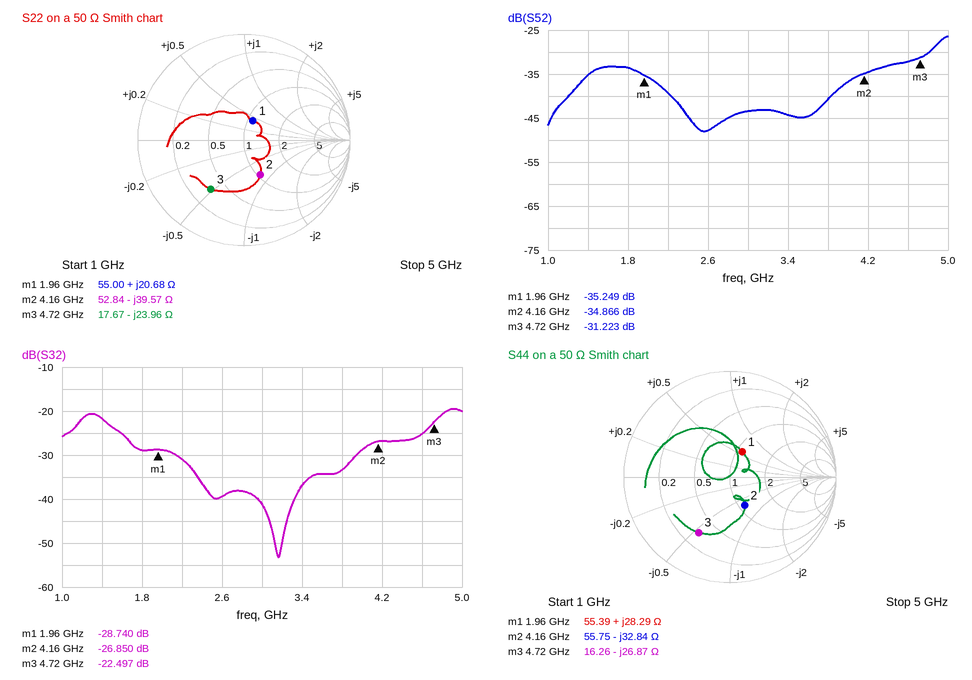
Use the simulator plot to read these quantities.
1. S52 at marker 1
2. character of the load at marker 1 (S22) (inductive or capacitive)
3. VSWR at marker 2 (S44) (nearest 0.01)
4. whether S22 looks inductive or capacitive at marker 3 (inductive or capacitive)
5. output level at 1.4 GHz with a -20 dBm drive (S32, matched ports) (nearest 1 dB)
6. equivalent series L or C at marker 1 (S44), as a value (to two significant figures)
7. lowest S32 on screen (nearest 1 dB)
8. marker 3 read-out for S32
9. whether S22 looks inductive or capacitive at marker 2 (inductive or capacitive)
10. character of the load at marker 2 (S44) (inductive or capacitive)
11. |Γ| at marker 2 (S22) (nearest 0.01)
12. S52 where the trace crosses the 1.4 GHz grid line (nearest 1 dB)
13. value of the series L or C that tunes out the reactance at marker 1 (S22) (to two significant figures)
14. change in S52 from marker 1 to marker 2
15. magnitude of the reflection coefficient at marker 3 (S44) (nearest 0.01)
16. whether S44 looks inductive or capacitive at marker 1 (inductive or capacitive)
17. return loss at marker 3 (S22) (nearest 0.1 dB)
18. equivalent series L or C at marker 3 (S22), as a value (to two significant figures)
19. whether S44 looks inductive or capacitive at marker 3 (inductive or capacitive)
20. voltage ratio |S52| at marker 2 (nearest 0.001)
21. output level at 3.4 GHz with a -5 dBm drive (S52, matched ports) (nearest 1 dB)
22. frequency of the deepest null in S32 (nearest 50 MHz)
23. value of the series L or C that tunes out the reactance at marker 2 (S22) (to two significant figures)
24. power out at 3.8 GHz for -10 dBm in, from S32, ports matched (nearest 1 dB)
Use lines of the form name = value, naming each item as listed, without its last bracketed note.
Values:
S52 at marker 1 = -35.249 dB
character of the load at marker 1 (S22) = inductive
VSWR at marker 2 (S44) = 1.86
whether S22 looks inductive or capacitive at marker 3 = capacitive
output level at 1.4 GHz with a -20 dBm drive (S32, matched ports) = -42 dBm
equivalent series L or C at marker 1 (S44), as a value = 2.3 nH
lowest S32 on screen = -53 dB
marker 3 read-out for S32 = -22.497 dB
whether S22 looks inductive or capacitive at marker 2 = capacitive
character of the load at marker 2 (S44) = capacitive
|Γ| at marker 2 (S22) = 0.36
S52 where the trace crosses the 1.4 GHz grid line = -35 dB
value of the series L or C that tunes out the reactance at marker 1 (S22) = 3.9 pF
change in S52 from marker 1 to marker 2 = 0.383 dB
magnitude of the reflection coefficient at marker 3 (S44) = 0.60
whether S44 looks inductive or capacitive at marker 1 = inductive
return loss at marker 3 (S22) = 5.0 dB
equivalent series L or C at marker 3 (S22), as a value = 1.4 pF
whether S44 looks inductive or capacitive at marker 3 = capacitive
voltage ratio |S52| at marker 2 = 0.018
output level at 3.4 GHz with a -5 dBm drive (S52, matched ports) = -49 dBm
frequency of the deepest null in S32 = 3.15 GHz
value of the series L or C that tunes out the reactance at marker 2 (S22) = 1.5 nH
power out at 3.8 GHz for -10 dBm in, from S32, ports matched = -43 dBm
